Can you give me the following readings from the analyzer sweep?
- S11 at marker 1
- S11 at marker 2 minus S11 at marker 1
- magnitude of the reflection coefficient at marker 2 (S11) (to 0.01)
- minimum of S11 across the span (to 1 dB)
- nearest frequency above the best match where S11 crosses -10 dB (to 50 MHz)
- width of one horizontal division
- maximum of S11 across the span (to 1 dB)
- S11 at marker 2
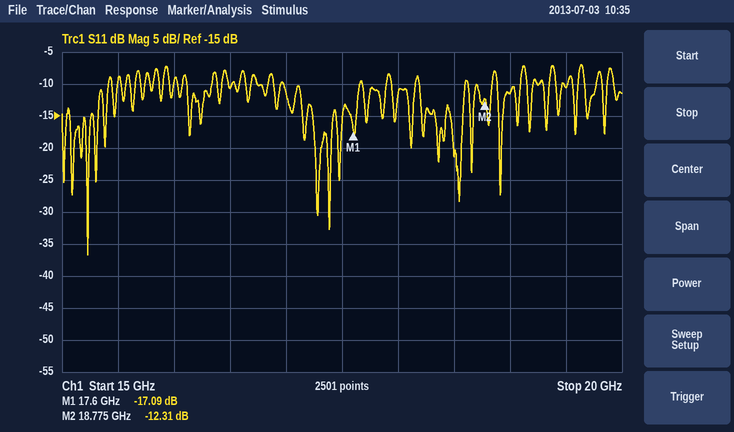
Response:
-17.09 dB
4.78 dB
0.24
-37 dB
15.40 GHz
500 MHz
-7 dB
-12.31 dB
